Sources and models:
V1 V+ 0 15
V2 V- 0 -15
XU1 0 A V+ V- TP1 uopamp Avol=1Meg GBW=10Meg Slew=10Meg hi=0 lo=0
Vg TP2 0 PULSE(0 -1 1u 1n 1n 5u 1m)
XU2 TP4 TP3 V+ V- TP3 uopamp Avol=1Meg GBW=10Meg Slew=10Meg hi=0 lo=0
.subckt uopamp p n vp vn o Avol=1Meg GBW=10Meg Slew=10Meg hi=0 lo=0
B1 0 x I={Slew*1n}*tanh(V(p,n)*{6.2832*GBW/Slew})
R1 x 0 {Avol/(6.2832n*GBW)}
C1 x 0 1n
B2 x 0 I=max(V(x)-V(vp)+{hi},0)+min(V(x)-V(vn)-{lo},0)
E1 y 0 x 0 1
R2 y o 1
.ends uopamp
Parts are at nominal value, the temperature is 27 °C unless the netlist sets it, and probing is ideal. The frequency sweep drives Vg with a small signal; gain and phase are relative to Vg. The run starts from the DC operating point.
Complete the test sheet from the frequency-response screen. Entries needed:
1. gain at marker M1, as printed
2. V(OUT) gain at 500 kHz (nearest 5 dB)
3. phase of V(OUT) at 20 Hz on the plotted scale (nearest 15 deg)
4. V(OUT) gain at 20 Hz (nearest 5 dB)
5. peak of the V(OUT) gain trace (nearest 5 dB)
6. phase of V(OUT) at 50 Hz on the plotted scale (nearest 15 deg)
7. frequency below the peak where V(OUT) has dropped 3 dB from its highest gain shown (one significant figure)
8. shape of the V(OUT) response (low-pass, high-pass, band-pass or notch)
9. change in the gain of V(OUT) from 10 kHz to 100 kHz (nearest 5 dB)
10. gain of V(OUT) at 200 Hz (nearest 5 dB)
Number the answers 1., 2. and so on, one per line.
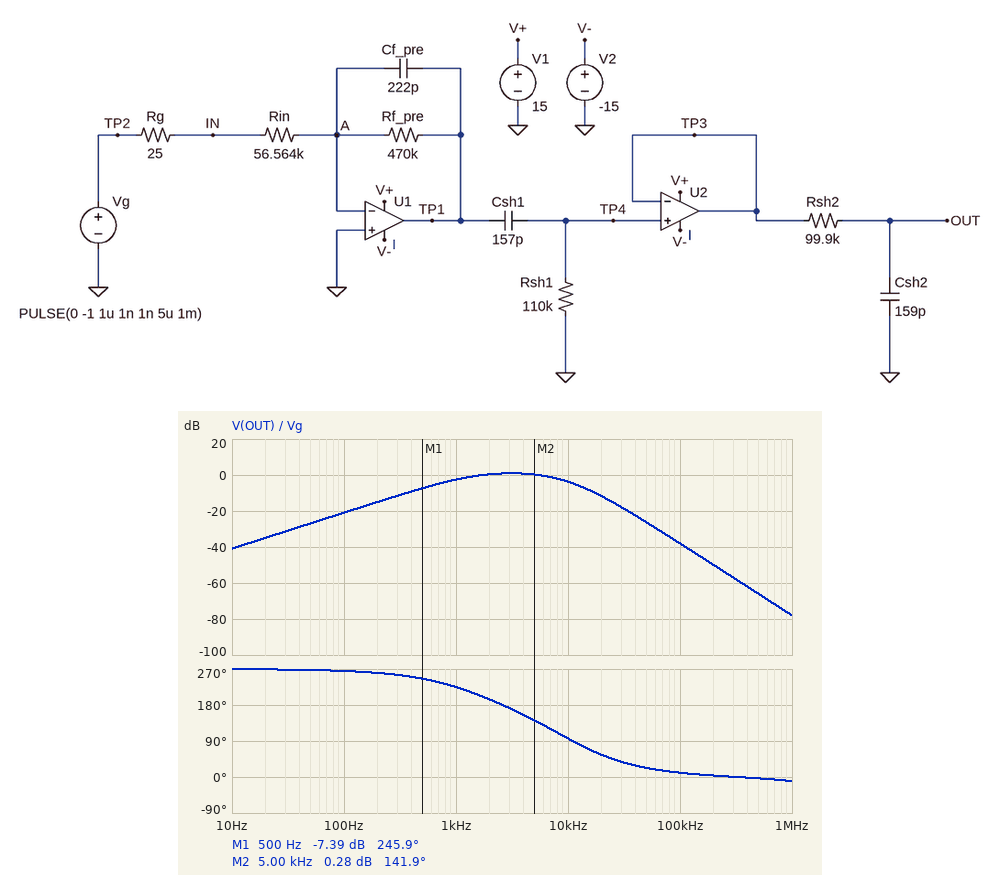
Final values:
1. -7.39 dB
2. -65 dB
3. 270 deg
4. -35 dB
5. 0 dB
6. 270 deg
7. 1 kHz
8. band-pass
9. -35 dB
10. -15 dB
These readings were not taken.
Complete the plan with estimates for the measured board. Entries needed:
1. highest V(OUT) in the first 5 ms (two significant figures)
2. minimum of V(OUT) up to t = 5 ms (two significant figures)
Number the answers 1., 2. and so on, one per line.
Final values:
1. 140 mV
2. -28 mV
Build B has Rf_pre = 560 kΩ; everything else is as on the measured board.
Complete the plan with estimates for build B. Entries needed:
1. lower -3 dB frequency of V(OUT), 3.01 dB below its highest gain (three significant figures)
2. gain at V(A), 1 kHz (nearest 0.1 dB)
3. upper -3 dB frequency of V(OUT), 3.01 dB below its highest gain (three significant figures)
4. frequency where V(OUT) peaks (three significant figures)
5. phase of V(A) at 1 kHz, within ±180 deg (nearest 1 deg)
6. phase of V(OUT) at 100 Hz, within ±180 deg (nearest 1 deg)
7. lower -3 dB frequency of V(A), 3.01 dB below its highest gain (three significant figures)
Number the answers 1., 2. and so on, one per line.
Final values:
1. 956 Hz
2. -62.2 dB
3. 7.83 kHz
4. 2.88 kHz
5. 51 deg
6. -96 deg
7. 1.28 kHz
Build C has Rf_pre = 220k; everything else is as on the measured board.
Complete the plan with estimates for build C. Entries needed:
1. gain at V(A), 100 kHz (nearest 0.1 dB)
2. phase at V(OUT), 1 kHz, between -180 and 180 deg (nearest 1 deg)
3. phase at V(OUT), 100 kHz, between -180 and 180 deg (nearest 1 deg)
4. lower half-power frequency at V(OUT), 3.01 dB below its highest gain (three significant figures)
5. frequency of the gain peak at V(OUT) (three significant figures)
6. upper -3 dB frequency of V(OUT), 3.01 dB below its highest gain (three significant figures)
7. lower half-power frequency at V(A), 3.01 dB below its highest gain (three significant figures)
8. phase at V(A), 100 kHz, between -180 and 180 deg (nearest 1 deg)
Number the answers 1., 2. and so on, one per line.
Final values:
1. -58.0 dB
2. -119 deg
3. 12 deg
4. 1.81 kHz
5. 4.43 kHz
6. 9.69 kHz
7. 3.25 kHz
8. 1 deg
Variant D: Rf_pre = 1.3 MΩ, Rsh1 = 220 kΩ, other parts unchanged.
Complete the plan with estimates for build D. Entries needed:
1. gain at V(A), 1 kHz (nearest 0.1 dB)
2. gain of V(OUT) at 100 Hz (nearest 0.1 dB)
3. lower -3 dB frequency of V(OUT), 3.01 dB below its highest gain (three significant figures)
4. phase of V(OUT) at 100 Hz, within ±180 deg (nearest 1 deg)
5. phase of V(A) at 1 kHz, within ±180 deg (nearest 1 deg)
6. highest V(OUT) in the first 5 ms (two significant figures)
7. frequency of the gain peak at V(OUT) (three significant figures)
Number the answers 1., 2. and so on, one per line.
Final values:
1. -59.1 dB
2. -6.2 dB
3. 444 Hz
4. -102 deg
5. 28 deg
6. 190 mV
7. 1.50 kHz
